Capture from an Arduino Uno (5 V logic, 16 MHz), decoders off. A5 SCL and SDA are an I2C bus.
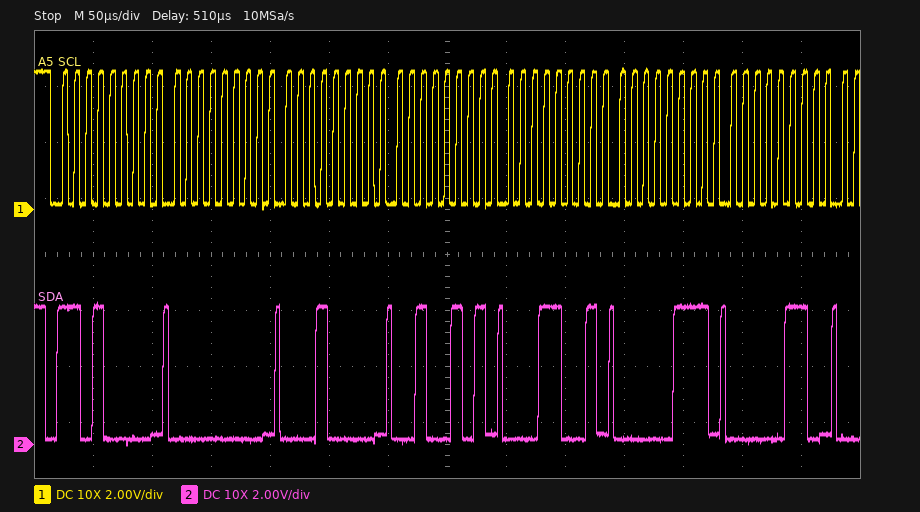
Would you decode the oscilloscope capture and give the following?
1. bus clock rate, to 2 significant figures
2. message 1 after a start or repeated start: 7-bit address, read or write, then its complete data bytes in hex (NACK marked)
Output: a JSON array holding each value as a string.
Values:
["100 kHz", "0x68 write: 00 10 25 19 07 06"]
